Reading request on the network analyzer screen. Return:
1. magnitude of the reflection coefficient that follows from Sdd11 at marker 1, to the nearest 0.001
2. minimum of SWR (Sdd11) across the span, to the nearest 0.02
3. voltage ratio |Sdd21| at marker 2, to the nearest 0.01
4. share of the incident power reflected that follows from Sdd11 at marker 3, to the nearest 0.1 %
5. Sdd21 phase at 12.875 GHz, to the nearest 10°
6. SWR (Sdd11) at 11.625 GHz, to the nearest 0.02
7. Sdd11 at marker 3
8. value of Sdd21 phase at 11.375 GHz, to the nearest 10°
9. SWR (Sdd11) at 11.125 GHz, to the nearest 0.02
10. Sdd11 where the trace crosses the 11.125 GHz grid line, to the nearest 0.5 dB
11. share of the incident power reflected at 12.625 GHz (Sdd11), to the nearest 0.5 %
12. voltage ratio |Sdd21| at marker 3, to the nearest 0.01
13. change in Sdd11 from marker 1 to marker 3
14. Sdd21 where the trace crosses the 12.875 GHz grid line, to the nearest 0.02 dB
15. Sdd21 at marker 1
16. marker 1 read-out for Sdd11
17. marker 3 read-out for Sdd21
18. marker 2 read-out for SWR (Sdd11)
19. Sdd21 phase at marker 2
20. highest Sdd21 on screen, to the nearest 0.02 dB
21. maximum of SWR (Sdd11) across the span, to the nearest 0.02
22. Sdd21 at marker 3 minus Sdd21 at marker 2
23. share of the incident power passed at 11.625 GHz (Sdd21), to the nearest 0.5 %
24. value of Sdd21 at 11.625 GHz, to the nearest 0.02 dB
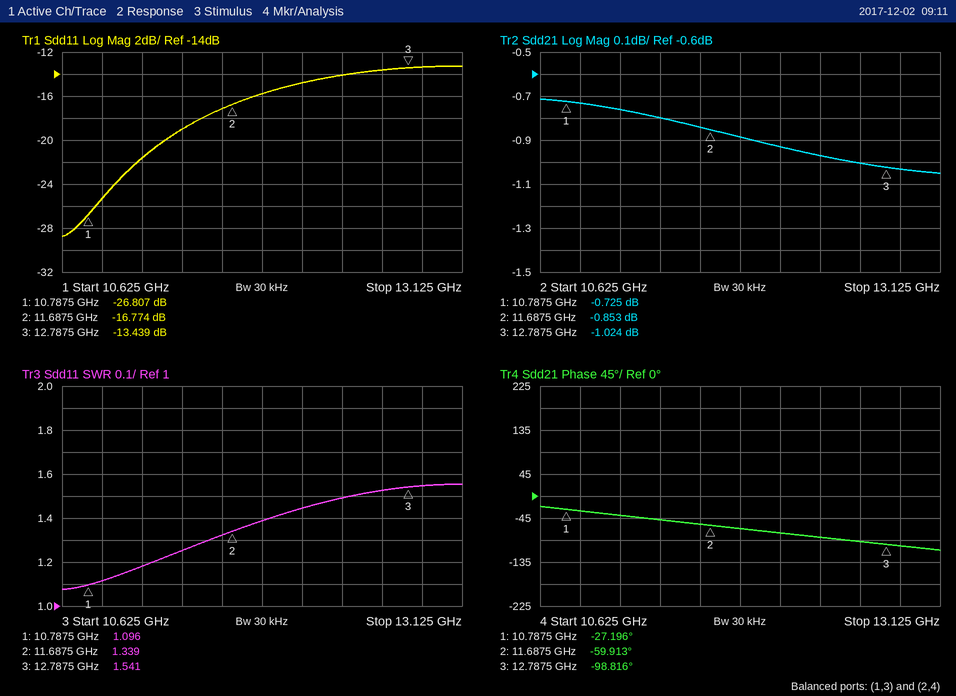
0.046
1.08
0.91
4.5 %
-100°
1.32
-13.439 dB
-50°
1.18
-21.5 dB
4.5 %
0.89
13.368 dB
-1.04 dB
-0.725 dB
-26.807 dB
-1.024 dB
1.339
-59.913°
-0.72 dB
1.56
-0.171 dB
82.5 %
-0.84 dB
